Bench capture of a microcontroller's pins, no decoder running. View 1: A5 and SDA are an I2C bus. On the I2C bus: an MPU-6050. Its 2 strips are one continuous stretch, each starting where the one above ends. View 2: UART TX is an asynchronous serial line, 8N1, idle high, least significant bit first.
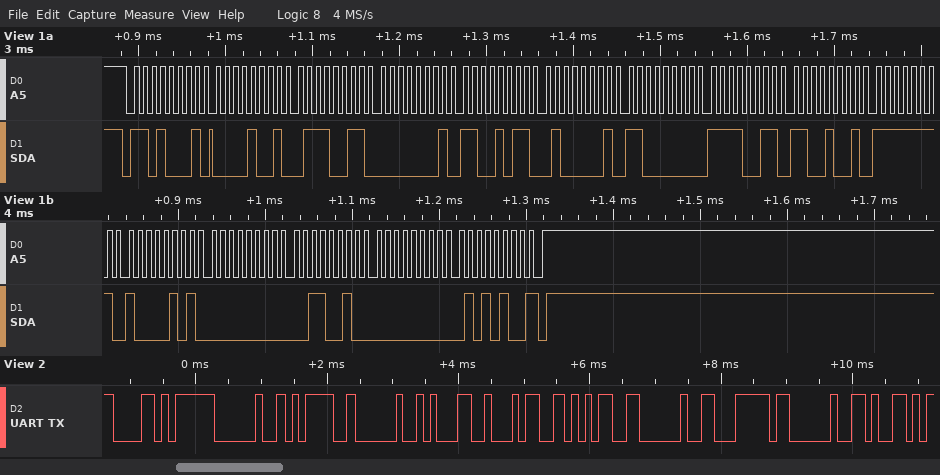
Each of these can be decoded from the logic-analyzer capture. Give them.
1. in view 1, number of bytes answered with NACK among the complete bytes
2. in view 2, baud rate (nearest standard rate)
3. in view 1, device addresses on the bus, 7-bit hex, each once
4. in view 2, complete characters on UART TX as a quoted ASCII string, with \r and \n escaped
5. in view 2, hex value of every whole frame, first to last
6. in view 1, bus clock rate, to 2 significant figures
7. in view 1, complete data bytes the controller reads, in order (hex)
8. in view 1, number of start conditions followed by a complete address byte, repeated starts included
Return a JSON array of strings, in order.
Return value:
["1", "9600 baud", "0x68", "\"X = 145 | Y\"", "0x58 0x20 0x3D 0x20 0x31 0x34 0x35 0x20 0x7C 0x20 0x59", "100 kHz", "09 73 01 CB 41 C0 F3 C9 FF 85 00 32 00 54", "1"]
